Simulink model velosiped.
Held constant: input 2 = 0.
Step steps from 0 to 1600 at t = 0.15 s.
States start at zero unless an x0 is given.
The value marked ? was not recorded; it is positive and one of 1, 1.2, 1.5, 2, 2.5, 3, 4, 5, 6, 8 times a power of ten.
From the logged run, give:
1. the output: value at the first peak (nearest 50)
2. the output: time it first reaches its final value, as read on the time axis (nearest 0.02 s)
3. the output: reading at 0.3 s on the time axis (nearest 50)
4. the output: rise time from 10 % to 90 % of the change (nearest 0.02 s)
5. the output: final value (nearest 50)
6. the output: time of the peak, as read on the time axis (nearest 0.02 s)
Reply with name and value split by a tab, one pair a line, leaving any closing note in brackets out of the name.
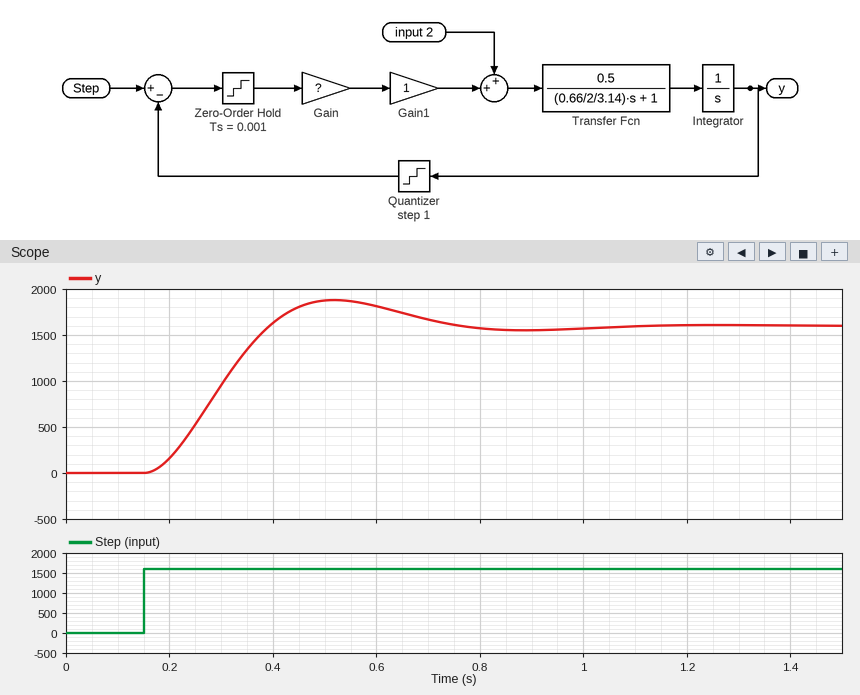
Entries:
the output: value at the first peak	1900
the output: time it first reaches its final value, as read on the time axis	0.40 s
the output: reading at 0.3 s on the time axis	950
the output: rise time from 10 % to 90 % of the change	0.16 s
the output: final value	1600
the output: time of the peak, as read on the time axis	0.52 s
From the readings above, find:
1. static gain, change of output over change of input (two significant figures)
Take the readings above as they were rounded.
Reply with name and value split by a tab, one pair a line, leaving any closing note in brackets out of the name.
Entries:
static gain, change of output over change of input	1.0
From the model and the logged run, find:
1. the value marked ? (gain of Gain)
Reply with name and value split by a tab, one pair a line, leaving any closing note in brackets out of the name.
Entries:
the value marked ?	20
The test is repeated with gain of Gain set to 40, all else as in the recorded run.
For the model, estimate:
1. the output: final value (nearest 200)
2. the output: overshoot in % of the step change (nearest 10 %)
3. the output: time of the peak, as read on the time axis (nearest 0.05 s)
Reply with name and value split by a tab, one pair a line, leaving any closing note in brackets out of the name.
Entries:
the output: final value	1600
the output: overshoot in % of the step change	30 %
the output: time of the peak, as read on the time axis	0.40 s
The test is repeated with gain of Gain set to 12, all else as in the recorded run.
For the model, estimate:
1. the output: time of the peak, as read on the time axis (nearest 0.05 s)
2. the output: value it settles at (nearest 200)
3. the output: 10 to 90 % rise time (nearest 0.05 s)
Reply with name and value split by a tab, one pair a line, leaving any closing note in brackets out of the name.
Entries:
the output: time of the peak, as read on the time axis	0.70 s
the output: value it settles at	1600
the output: 10 to 90 % rise time	0.25 s
